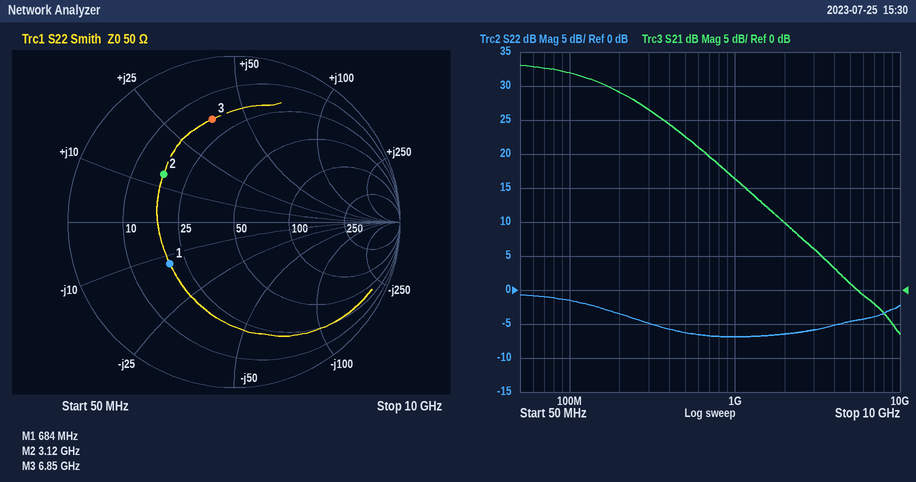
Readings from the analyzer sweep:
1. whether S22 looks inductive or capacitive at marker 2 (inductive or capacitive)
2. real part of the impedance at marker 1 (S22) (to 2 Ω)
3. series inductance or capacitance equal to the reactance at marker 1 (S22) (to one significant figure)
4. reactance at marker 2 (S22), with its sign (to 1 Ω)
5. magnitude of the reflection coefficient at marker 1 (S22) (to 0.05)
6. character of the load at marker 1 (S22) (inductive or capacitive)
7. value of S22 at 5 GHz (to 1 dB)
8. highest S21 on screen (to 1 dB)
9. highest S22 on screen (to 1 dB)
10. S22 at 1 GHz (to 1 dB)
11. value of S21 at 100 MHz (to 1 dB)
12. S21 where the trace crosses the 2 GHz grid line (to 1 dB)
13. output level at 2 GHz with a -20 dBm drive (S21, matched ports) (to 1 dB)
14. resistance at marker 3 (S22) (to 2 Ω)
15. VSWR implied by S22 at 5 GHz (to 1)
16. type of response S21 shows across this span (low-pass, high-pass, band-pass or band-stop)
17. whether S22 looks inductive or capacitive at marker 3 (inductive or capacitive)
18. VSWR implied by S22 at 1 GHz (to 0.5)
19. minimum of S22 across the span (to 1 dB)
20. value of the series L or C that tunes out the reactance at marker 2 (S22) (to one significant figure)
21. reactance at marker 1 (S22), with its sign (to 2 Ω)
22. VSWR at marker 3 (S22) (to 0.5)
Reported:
inductive
20 Ω
20 pF
+14 Ω
0.45
capacitive
-5 dB
33 dB
-1 dB
-7 dB
32 dB
10 dB
-10 dBm
18 Ω
4
low-pass
inductive
2.5
-7 dB
4 pF
-12 Ω
4.5
